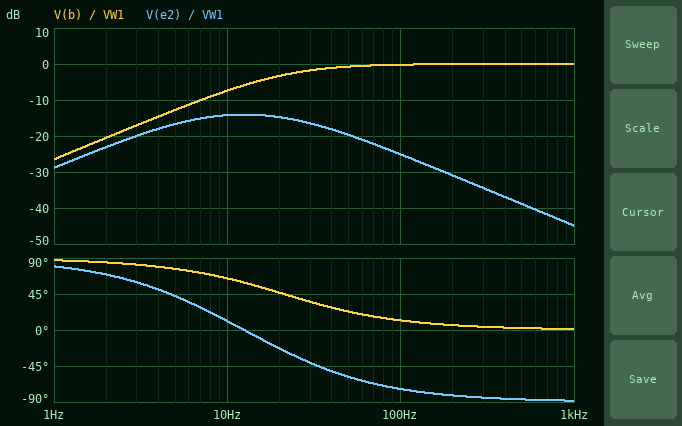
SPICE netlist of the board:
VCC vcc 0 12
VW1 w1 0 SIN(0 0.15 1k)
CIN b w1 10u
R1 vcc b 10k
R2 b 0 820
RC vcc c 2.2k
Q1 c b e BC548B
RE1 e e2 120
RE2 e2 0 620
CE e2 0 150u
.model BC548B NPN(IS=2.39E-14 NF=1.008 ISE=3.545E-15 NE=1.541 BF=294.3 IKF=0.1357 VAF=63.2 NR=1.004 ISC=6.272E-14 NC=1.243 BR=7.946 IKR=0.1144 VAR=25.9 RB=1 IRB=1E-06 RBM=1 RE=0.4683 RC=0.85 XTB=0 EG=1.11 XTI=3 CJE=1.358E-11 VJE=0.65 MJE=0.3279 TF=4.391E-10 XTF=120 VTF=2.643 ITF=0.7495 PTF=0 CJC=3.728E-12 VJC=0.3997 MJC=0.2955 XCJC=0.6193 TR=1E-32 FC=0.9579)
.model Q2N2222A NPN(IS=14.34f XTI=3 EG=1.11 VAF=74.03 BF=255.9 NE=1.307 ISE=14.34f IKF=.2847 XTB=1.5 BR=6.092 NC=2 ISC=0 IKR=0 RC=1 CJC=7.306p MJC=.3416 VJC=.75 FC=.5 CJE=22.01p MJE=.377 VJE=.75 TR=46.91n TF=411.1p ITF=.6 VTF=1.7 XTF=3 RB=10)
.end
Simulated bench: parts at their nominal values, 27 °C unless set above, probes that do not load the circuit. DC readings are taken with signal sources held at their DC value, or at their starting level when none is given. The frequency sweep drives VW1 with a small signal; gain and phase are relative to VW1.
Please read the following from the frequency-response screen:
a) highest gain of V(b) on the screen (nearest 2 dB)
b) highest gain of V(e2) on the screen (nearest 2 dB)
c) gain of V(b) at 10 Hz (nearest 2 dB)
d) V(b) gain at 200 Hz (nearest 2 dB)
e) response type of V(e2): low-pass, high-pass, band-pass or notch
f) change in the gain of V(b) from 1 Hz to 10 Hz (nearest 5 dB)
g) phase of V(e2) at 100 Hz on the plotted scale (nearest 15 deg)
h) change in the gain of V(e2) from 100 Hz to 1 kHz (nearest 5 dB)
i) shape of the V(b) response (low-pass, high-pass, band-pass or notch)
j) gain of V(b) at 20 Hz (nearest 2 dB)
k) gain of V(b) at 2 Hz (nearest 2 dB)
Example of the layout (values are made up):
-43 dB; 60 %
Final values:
0 dB; -14 dB; -8 dB; 0 dB; band-pass; 20 dB; -75 deg; -20 dB; high-pass; -4 dB; -20 dB
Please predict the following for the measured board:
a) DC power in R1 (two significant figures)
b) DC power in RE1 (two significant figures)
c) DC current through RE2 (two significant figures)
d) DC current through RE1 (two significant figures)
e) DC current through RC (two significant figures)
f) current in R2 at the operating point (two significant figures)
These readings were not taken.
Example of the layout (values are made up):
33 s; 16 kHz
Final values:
12 mW; 19 µW; 400 µA; 400 µA; 400 µA; 1.1 mA
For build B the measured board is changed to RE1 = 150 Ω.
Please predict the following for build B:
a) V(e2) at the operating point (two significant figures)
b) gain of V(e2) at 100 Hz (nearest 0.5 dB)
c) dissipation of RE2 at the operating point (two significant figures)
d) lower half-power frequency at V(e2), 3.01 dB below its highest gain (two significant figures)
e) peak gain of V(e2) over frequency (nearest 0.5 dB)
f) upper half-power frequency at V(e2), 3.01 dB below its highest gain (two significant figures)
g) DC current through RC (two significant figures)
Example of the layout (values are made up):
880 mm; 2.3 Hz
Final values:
240 mV; -26.5 dB; 93 µW; 4.3 Hz; -15.0 dB; 32 Hz; 390 µA
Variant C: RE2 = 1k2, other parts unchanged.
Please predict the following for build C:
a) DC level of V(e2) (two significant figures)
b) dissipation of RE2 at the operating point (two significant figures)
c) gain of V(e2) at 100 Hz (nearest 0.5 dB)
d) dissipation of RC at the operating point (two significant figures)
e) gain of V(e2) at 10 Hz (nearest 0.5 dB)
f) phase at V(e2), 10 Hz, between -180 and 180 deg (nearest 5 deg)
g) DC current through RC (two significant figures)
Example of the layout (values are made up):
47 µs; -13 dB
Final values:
280 mV; 67 µW; -27.0 dB; 120 µW; -15.5 dB; 5 deg; 240 µA
